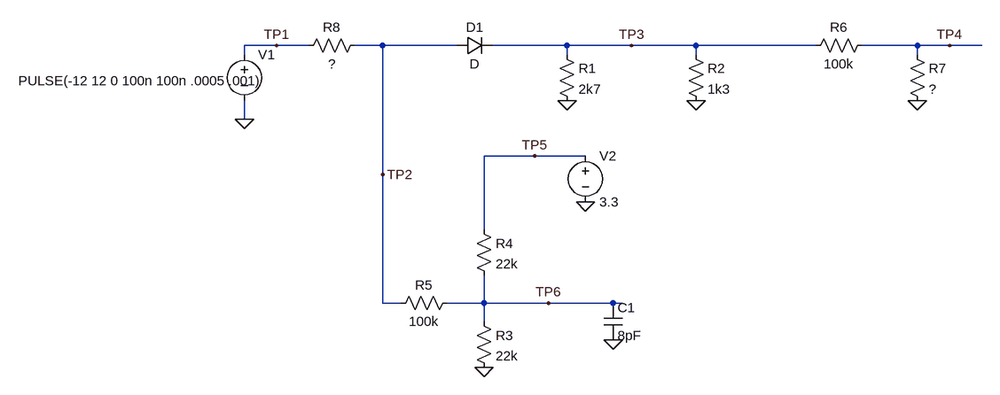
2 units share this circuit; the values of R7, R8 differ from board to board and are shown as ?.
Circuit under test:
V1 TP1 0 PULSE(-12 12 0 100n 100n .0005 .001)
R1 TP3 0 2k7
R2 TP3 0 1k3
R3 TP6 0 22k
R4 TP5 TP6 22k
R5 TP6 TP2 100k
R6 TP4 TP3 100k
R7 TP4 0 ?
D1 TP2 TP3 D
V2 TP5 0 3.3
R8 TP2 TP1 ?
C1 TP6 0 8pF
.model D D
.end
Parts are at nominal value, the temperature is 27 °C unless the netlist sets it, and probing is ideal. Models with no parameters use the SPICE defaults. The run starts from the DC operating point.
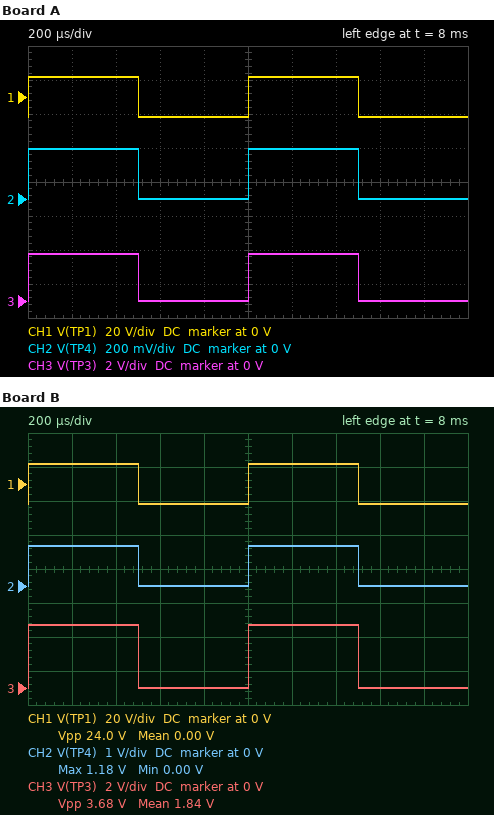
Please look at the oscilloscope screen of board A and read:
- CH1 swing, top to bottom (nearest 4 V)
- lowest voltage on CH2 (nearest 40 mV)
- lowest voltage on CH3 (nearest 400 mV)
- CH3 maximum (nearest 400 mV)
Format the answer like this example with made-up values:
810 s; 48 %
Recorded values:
24 V; 0 V; 0 V; 2.8 V
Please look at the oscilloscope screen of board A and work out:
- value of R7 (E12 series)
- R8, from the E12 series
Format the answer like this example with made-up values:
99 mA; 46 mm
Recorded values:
12 kΩ; 2.7 kΩ
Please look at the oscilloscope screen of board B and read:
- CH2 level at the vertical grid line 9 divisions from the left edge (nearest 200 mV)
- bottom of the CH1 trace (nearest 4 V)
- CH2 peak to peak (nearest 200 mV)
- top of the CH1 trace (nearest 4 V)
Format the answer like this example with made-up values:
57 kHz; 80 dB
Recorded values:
0 V; -12 V; 1.2 V; 12 V
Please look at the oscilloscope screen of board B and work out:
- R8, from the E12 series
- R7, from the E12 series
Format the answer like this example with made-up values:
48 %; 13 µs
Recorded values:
1.8 kΩ; 47 kΩ
